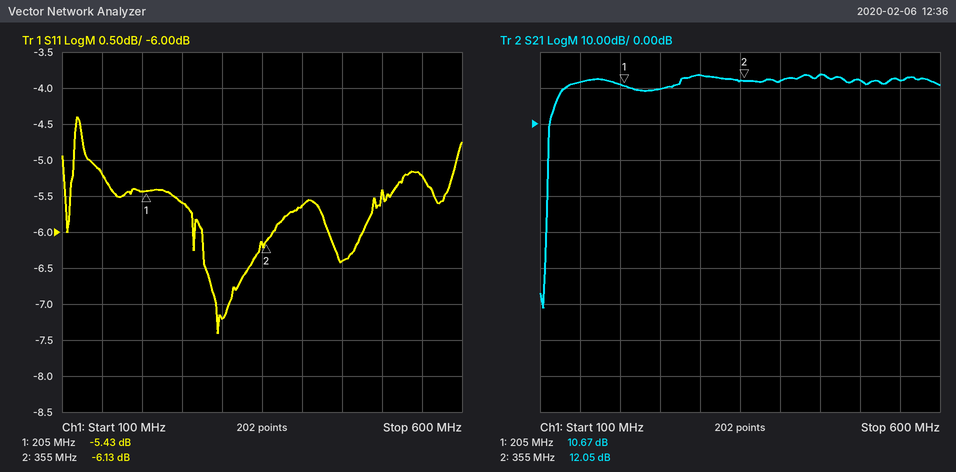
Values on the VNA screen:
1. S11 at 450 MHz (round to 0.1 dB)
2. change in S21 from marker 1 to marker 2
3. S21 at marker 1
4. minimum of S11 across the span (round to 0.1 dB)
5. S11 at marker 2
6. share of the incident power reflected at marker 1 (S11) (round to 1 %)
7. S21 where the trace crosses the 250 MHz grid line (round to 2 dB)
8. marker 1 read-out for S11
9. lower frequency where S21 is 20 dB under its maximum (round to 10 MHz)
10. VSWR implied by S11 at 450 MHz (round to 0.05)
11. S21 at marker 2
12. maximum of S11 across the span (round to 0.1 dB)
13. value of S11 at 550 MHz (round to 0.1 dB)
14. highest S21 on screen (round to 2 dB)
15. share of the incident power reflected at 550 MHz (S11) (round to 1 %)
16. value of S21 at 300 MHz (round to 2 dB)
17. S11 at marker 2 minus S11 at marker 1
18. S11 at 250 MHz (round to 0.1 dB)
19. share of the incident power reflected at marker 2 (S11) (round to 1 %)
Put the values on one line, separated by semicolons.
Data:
-6.4 dB; 1.38 dB; 10.67 dB; -7.4 dB; -6.13 dB; 29 %; 10 dB; -5.43 dB; 110 MHz; 2.85; 12.05 dB; -4.4 dB; -5.2 dB; 14 dB; 30 %; 14 dB; -0.70 dB; -5.6 dB; 24 %
